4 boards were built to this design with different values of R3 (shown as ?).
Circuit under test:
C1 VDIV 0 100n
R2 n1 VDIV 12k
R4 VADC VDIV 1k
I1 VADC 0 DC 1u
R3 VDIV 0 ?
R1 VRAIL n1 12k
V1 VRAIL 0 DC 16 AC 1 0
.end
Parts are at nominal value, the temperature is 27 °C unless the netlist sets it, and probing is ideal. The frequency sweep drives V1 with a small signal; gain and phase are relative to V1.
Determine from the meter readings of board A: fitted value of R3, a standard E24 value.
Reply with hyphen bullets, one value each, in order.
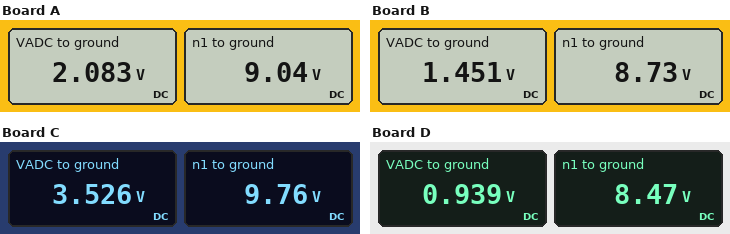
- 3.6 kΩ
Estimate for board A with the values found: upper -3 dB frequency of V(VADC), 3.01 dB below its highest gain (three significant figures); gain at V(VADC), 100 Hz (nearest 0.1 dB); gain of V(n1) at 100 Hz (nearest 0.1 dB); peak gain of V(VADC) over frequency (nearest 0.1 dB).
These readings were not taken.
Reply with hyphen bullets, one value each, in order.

- 508 Hz
- -17.9 dB
- -5.0 dB
- -17.7 dB
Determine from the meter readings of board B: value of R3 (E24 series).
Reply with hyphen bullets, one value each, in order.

- 2.4 kΩ
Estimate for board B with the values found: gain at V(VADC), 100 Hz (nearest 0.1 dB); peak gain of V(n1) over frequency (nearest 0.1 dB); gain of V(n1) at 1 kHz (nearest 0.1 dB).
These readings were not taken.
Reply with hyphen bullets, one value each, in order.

- -20.9 dB
- -5.3 dB
- -5.7 dB
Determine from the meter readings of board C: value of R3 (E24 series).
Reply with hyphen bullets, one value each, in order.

- 6.8 kΩ
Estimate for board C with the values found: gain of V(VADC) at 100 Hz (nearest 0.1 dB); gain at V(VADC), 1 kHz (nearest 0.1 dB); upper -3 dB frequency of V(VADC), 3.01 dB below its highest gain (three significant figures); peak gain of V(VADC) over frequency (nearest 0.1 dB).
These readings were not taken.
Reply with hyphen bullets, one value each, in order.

- -13.6 dB
- -23.9 dB
- 300 Hz
- -13.1 dB
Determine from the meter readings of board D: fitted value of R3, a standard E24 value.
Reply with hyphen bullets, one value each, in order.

- 1.5 kΩ
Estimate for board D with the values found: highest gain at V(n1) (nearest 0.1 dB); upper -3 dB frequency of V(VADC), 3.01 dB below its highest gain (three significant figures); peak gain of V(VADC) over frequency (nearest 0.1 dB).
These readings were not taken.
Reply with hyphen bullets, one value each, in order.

- -5.5 dB
- 1.13 kHz
- -24.6 dB
